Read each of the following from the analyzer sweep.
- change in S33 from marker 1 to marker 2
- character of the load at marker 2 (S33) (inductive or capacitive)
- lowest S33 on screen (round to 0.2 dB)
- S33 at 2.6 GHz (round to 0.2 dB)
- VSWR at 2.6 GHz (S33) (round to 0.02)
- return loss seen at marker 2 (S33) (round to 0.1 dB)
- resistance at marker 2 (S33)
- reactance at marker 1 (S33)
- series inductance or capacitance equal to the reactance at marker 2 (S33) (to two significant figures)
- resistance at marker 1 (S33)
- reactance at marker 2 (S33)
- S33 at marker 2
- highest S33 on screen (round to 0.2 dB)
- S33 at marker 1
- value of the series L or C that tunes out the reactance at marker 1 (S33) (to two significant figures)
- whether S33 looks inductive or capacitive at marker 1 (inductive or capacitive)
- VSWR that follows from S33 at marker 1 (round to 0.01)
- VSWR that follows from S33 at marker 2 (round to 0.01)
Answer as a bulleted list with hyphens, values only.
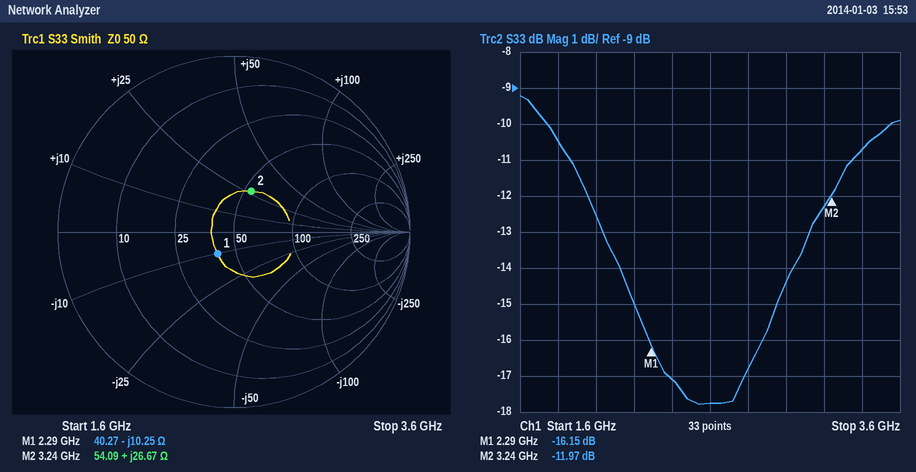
- 4.18 dB
- inductive
- -17.8 dB
- -17.8 dB
- 1.30
- 12.0 dB
- 54.09 Ω
- -10.25 Ω
- 1.3 nH
- 40.27 Ω
- +26.67 Ω
- -11.97 dB
- -9.2 dB
- -16.15 dB
- 710 pH
- capacitive
- 1.37
- 1.67
